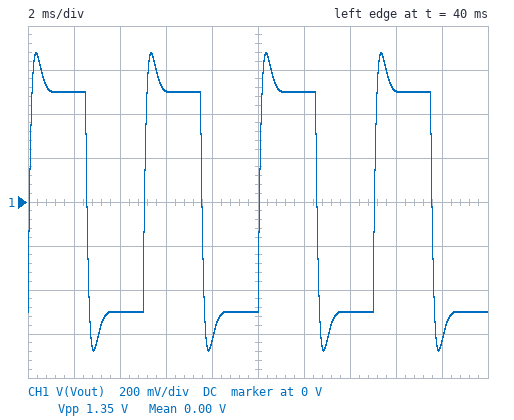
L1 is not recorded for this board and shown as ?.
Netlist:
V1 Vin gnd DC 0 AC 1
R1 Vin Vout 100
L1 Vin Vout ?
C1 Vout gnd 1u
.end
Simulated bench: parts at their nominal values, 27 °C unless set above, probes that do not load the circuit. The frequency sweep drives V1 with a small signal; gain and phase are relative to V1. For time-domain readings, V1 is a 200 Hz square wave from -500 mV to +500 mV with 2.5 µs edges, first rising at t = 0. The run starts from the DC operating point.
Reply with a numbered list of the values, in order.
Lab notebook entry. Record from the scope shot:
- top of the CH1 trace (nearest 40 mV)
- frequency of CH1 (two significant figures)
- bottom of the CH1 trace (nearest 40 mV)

1. 680 mV
2. 200 Hz
3. -680 mV
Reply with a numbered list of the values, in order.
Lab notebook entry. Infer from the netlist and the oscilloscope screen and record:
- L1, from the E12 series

1. 27 mH
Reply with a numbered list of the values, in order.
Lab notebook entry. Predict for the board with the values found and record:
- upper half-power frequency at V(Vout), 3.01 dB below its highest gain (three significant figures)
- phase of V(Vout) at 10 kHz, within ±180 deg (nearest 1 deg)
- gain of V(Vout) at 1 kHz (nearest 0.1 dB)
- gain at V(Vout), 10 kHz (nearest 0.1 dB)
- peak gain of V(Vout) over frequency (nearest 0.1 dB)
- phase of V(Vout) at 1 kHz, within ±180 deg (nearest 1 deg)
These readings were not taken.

1. 1.70 kHz
2. -84 deg
3. 1.3 dB
4. -16.0 dB
5. 1.7 dB
6. -33 deg
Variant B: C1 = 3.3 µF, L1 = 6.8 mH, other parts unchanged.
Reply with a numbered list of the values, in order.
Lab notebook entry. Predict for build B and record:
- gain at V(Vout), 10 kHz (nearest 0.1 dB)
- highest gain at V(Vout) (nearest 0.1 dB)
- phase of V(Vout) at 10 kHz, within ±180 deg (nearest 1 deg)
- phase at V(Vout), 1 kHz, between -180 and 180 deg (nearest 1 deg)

1. -26.0 dB
2. 7.8 dB
3. -100 deg
4. -52 deg
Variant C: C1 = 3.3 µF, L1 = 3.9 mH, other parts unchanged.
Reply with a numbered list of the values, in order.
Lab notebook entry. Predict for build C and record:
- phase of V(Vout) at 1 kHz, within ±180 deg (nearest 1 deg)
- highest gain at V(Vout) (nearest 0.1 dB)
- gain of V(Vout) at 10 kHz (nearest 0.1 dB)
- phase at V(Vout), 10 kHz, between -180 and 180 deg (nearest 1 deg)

1. -13 deg
2. 9.9 dB
3. -25.5 dB
4. -109 deg
